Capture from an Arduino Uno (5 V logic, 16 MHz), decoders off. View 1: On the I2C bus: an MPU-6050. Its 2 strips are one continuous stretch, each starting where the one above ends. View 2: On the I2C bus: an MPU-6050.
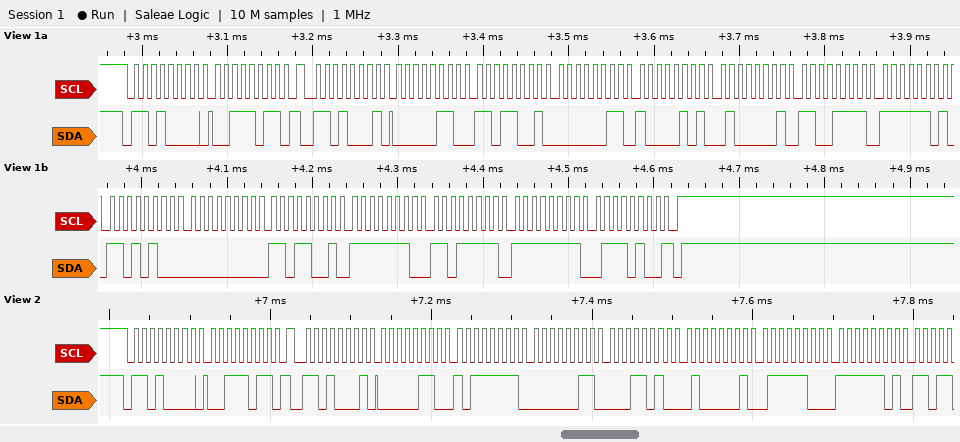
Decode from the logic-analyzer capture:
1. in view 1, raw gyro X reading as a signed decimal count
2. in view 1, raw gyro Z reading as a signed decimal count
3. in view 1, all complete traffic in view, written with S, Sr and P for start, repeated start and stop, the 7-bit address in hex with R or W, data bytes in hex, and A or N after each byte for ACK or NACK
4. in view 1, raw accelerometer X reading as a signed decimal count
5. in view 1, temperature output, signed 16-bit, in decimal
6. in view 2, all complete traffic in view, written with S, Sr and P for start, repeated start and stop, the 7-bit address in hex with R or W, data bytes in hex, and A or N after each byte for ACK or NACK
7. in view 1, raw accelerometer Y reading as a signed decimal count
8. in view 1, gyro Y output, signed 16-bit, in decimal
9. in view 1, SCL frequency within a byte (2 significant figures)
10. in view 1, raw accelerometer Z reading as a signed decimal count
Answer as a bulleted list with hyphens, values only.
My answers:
- 217
- -140
- S 68W A 3B A Sr 68R A 06 A D9 A 03 A 85 A 41 A CF A FD A D4 A 00 A D9 A FE A DF A FF A 74 N P
- 1753
- -556
- S 68W A 3B A Sr 68R A 06 A BF A 03 A 1A A 41 A 7C A FD A
- 901
- -289
- 100 kHz
- 16847
